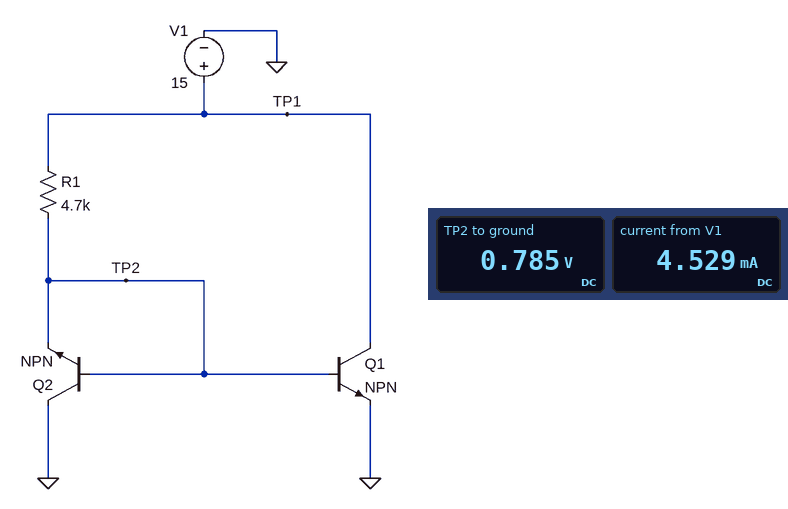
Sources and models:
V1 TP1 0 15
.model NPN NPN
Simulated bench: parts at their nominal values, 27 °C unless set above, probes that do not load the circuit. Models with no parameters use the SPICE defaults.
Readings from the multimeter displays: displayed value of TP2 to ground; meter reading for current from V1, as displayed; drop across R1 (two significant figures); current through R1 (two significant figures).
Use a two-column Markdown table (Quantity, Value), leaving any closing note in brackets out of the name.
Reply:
| Quantity | Value |
|---|---|
| displayed value of TP2 to ground | 0.785 V |
| meter reading for current from V1, as displayed | 4.529 mA |
| drop across R1 | 14 V |
| current through R1 | 3.0 mA |
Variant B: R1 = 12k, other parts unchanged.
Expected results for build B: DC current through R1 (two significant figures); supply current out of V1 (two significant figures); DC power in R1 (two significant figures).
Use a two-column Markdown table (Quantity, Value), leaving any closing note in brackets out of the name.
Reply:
| Quantity | Value |
|---|---|
| DC current through R1 | 1.2 mA |
| supply current out of V1 | 1.8 mA |
| DC power in R1 | 17 mW |
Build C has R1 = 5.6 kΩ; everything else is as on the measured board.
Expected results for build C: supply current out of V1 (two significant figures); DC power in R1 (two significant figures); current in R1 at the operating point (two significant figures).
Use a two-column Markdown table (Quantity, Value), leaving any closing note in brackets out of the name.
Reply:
| Quantity | Value |
|---|---|
| supply current out of V1 | 3.8 mA |
| DC power in R1 | 36 mW |
| current in R1 at the operating point | 2.5 mA |
